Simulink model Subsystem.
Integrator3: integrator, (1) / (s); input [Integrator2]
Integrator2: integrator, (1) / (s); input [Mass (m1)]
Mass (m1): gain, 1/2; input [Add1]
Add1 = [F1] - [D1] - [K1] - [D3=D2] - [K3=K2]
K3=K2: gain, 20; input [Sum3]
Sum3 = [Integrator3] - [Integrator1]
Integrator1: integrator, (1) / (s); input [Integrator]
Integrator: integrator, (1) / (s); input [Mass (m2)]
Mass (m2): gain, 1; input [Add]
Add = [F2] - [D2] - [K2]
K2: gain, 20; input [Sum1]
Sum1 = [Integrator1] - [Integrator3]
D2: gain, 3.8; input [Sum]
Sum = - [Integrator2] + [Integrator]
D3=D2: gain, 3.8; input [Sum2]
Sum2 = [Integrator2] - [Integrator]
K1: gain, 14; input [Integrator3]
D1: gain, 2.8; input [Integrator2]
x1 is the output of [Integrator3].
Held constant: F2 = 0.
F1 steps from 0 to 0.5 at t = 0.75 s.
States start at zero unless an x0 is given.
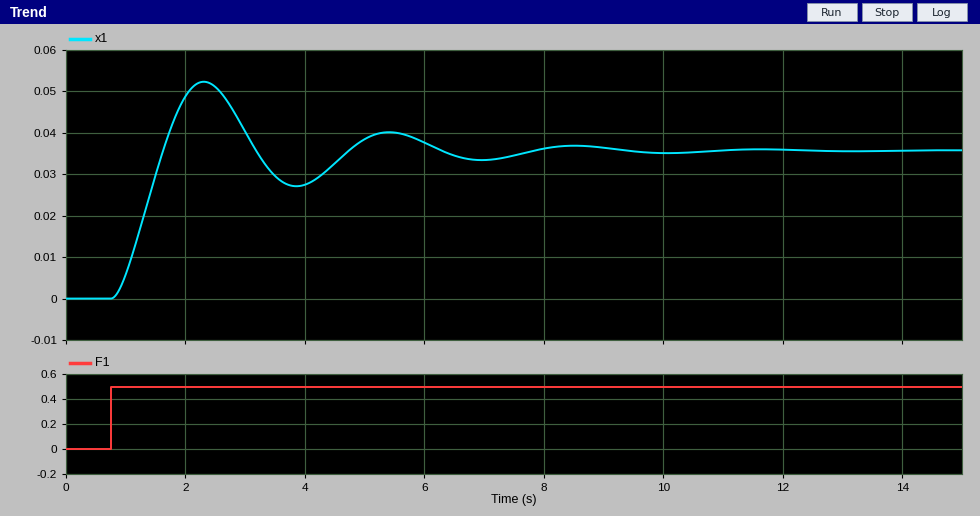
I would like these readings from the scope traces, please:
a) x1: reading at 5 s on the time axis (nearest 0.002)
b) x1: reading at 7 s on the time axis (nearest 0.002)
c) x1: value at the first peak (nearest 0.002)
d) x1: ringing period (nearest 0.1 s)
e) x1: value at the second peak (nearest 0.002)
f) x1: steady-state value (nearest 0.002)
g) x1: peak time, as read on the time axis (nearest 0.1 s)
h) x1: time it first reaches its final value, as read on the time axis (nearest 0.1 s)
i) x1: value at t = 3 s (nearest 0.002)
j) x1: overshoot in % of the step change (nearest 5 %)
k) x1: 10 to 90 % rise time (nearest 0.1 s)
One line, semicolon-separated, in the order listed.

0.038; 0.034; 0.052; 3.1 s; 0.040; 0.036; 2.3 s; 1.6 s; 0.040; 45 %; 0.6 s
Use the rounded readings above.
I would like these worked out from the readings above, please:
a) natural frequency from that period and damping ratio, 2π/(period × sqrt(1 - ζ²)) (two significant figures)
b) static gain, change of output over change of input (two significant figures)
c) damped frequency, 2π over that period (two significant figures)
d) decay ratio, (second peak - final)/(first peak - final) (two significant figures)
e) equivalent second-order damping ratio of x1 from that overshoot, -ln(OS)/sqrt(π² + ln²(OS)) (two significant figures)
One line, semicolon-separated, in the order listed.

2.1 rad/s; 0.072; 2.0 rad/s; 0.25; 0.25
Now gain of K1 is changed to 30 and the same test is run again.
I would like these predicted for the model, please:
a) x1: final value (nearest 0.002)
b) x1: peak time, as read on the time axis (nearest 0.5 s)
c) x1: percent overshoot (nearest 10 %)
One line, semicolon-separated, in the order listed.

0.016; 2.0 s; 50 %
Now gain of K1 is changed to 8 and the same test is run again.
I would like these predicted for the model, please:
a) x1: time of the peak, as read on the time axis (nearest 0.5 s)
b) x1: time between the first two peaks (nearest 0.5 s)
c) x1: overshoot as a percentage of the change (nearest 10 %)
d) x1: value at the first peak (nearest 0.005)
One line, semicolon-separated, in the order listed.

3.0 s; 4.0 s; 40 %; 0.085
